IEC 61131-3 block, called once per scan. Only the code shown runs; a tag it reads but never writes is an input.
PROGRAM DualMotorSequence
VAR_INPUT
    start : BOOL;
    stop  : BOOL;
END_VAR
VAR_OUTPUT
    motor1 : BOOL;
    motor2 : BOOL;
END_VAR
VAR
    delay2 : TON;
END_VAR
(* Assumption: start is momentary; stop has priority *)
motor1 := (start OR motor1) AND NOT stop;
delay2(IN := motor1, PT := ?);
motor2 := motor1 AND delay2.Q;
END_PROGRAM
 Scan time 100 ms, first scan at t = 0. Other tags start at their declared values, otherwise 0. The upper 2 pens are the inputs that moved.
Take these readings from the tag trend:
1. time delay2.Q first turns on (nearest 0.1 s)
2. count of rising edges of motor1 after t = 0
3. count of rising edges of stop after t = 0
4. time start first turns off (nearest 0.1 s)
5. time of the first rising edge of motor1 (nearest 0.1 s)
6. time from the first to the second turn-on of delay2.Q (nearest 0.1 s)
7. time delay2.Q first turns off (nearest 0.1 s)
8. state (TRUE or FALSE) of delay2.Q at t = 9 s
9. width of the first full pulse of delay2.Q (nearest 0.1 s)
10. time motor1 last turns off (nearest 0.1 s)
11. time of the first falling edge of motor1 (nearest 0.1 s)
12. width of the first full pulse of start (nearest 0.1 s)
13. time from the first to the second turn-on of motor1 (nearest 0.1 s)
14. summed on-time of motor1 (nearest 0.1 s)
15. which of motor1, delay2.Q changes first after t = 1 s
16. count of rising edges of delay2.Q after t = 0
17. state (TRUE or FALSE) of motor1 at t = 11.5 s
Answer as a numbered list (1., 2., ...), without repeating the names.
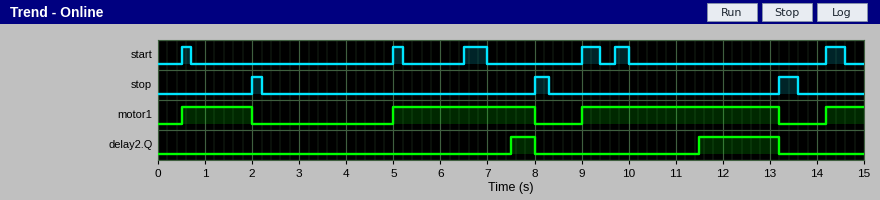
1. 7.5 s
2. 4
3. 3
4. 0.7 s
5. 0.5 s
6. 4.0 s
7. 8.0 s
8. FALSE
9. 0.5 s
10. 13.2 s
11. 2.0 s
12. 0.2 s
13. 4.5 s
14. 9.5 s
15. motor1
16. 2
17. TRUE
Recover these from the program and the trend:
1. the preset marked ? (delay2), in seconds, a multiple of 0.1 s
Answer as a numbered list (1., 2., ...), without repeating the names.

1. 2.5 s
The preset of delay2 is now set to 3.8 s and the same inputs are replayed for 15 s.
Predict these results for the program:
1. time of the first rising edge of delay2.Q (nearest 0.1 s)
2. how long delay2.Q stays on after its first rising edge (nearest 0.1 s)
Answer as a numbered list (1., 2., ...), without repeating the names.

1. 12.8 s
2. 0.4 s
